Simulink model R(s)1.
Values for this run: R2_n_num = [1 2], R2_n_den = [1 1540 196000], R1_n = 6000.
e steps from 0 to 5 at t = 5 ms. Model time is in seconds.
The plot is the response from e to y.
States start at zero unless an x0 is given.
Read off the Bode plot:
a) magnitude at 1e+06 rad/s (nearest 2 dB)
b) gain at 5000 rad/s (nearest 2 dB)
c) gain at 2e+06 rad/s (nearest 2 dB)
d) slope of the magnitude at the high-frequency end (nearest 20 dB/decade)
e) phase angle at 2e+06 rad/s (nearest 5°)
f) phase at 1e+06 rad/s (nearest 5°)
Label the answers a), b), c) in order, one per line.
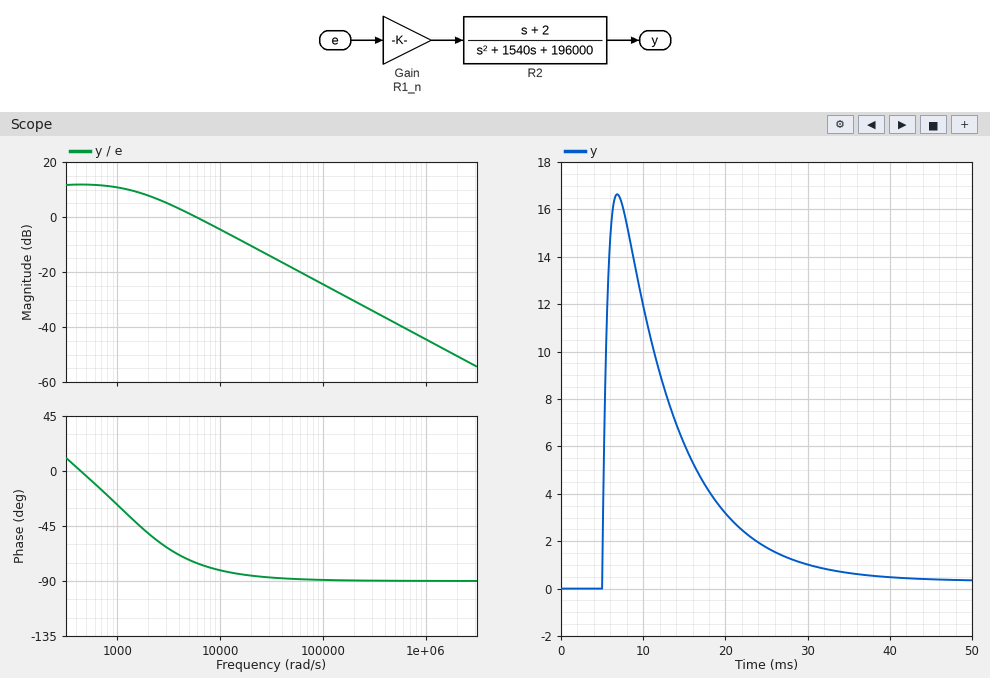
a) -44 dB
b) 2 dB
c) -50 dB
d) -20 dB/decade
e) -90°
f) -90°
